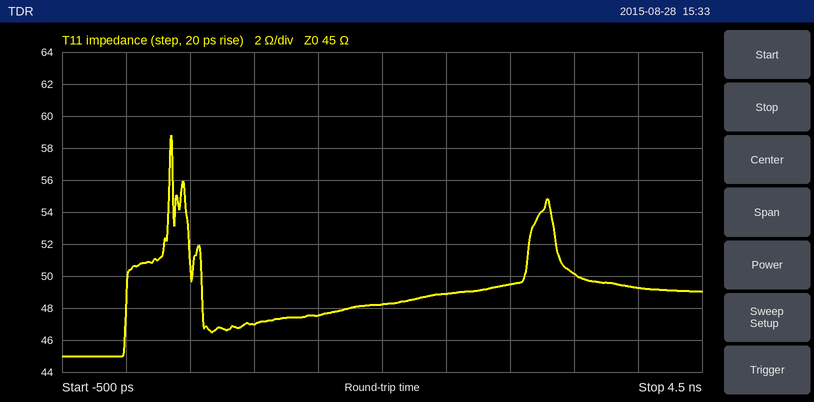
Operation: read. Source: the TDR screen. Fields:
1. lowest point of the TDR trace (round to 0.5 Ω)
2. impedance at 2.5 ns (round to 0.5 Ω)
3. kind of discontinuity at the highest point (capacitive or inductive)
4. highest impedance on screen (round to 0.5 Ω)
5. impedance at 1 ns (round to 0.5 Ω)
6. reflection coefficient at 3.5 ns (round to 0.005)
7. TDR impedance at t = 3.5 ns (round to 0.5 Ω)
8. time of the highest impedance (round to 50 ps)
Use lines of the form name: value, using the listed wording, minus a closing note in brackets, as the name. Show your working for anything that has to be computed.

lowest point of the TDR trace: 45.0 Ω
impedance at 2.5 ns: 49.0 Ω
kind of discontinuity at the highest point: inductive
highest impedance on screen: 59.0 Ω
impedance at 1 ns: 47.0 Ω
reflection coefficient at 3.5 ns: (50 − 45)/(50 + 45) ≈ +0.0526, so +0.055 to the nearest 0.005
TDR impedance at t = 3.5 ns: 50.0 Ω
time of the highest impedance: 350 ps
